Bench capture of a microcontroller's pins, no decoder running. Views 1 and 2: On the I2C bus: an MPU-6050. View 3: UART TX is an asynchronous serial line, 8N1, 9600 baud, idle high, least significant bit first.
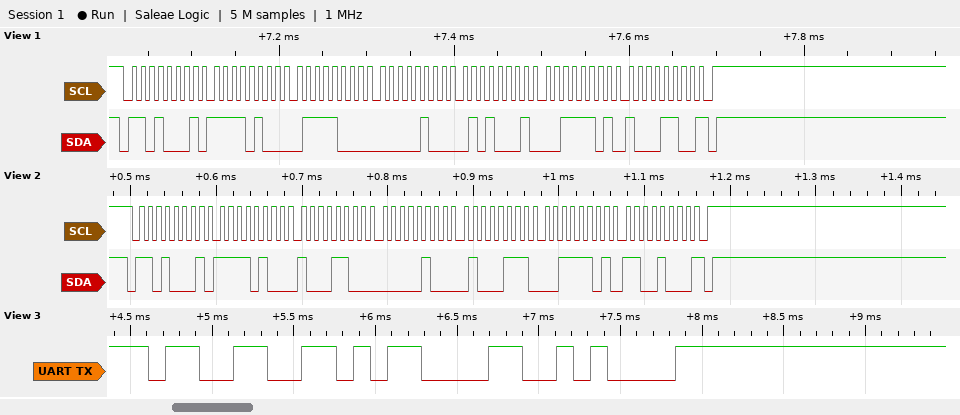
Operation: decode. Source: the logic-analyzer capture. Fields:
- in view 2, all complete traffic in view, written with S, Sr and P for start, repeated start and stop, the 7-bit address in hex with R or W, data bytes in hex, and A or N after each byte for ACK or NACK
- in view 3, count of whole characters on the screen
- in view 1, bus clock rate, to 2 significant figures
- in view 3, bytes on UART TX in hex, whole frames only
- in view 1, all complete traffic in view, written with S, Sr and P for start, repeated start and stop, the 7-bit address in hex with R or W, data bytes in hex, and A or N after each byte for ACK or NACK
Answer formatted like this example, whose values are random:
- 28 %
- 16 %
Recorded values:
- S 68R A F4 A 8C A 04 A 47 A 3D A C8 N P
- 3
- 100 kHz
- 0x33 0x0D 0x0A
- S 68R A F4 A 78 A 04 A 51 A 3D A 8C N P
